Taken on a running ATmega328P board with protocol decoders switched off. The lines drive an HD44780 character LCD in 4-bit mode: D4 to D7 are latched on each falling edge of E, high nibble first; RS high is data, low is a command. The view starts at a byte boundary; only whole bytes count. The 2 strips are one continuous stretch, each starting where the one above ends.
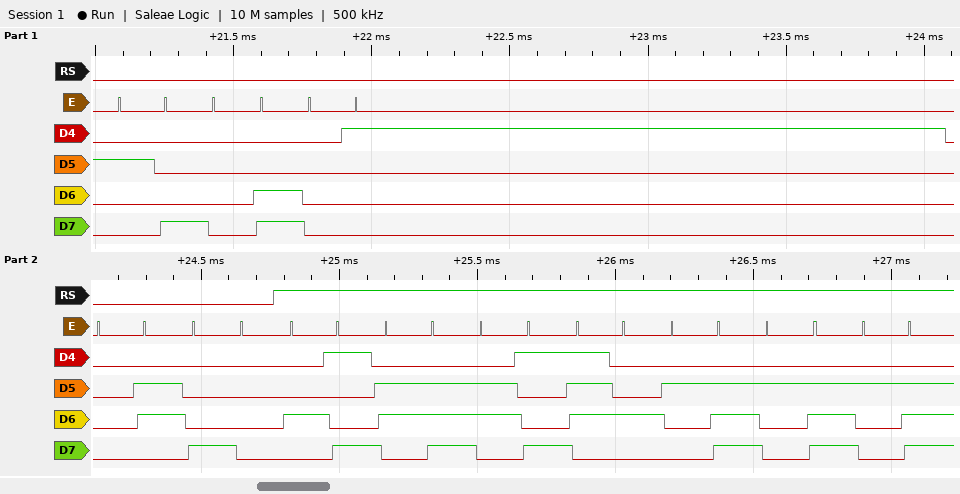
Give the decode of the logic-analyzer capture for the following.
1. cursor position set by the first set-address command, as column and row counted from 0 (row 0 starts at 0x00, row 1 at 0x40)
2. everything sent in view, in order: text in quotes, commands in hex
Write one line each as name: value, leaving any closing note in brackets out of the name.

cursor position set by the first set-address command, as column and row counted from 0: column 0, row 0
everything sent in view, in order: text in quotes, commands in hex: 0x28 0x0C 0x01 0x06 0x80 "Init..."
